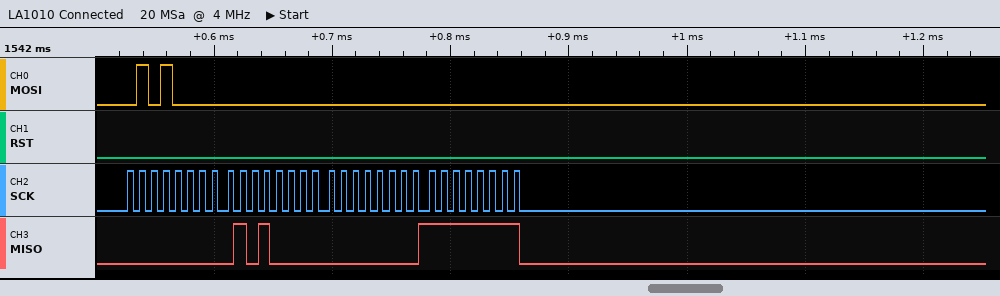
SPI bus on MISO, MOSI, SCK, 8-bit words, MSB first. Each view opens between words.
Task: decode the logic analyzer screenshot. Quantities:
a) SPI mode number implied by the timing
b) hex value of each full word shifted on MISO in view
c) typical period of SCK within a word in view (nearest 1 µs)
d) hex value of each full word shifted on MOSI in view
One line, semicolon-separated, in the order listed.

0; 00, 50, 00, FF; 10 µs; 50, 00, 00, 00
